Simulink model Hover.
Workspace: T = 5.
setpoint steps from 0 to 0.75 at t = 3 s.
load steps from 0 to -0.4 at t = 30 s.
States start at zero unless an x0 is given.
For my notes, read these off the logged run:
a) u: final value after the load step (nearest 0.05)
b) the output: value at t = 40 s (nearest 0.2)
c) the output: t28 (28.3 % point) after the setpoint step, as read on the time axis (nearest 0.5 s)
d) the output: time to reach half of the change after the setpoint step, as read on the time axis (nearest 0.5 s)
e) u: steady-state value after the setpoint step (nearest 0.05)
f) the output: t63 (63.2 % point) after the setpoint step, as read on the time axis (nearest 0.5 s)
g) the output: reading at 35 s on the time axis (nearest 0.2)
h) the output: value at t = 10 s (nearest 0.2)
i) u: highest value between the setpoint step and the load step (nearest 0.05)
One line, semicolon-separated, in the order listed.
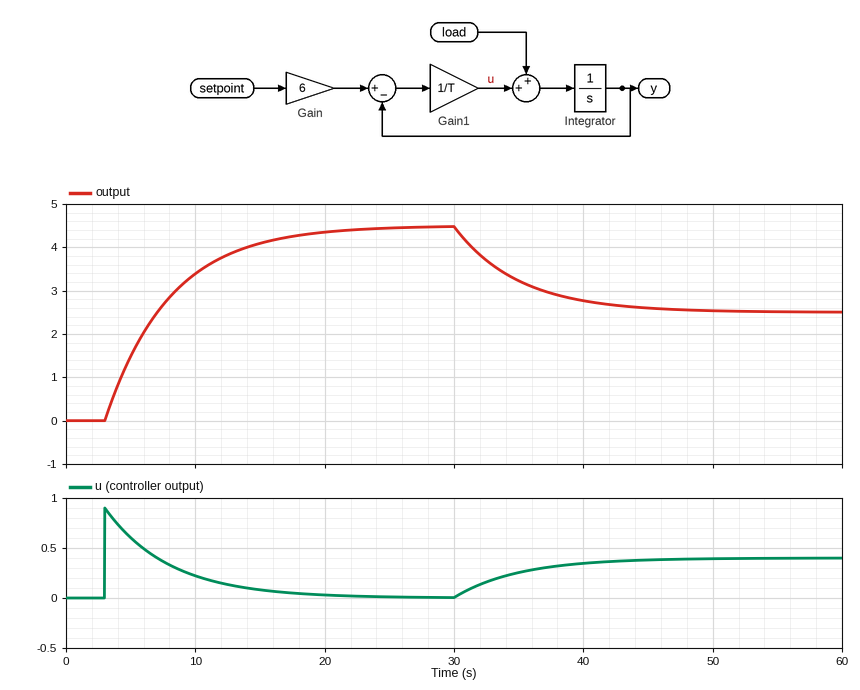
0.40; 2.8; 4.5 s; 6.5 s; 0.00; 8.0 s; 3.2; 3.4; 0.90
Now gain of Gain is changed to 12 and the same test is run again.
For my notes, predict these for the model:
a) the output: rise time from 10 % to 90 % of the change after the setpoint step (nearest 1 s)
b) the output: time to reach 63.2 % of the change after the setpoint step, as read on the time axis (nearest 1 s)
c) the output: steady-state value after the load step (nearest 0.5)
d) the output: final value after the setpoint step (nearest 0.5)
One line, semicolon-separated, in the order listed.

11 s; 8 s; 7.0; 9.0
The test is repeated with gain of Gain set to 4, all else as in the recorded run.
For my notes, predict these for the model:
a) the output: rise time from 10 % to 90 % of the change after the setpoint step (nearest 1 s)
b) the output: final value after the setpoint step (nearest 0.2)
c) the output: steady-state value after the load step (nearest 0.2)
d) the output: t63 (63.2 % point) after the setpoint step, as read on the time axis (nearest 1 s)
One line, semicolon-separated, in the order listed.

11 s; 3.0; 1.0; 8 s
